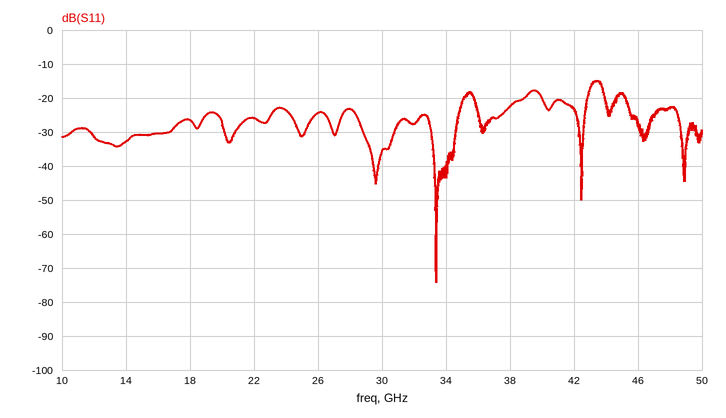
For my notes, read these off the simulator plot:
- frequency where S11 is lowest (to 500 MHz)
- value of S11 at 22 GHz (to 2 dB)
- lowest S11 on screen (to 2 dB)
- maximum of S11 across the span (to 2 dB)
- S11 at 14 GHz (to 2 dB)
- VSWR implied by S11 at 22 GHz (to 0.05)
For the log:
33.5 GHz
-26 dB
-74 dB
-14 dB
-32 dB
1.10
